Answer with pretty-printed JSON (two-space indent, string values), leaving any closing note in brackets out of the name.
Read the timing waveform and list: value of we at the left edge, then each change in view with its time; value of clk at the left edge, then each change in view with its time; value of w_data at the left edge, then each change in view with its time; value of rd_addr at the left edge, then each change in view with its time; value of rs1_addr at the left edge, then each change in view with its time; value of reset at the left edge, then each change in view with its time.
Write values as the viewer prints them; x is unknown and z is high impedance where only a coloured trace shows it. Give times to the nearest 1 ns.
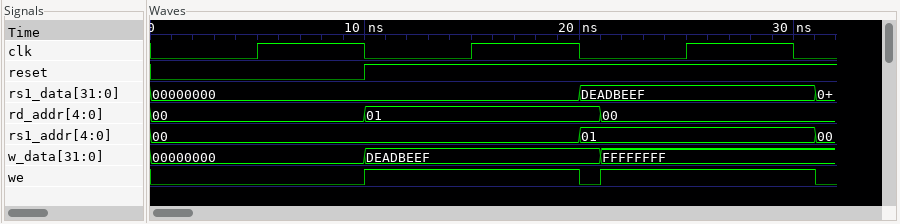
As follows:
{
  "value of we at the left edge, then each change in view with its time": "0, 1 at 10 ns, 0 at 20 ns, 1 at 21 ns, 0 at 31 ns",
  "value of clk at the left edge, then each change in view with its time": "0, 1 at 5 ns, 0 at 10 ns, 1 at 15 ns, 0 at 20 ns, 1 at 25 ns, 0 at 30 ns",
  "value of w_data at the left edge, then each change in view with its time": "00000000, DEADBEEF at 10 ns, FFFFFFFF at 21 ns",
  "value of rd_addr at the left edge, then each change in view with its time": "00, 01 at 10 ns, 00 at 21 ns",
  "value of rs1_addr at the left edge, then each change in view with its time": "00, 01 at 20 ns, 00 at 31 ns",
  "value of reset at the left edge, then each change in view with its time": "0, 1 at 10 ns"
}
